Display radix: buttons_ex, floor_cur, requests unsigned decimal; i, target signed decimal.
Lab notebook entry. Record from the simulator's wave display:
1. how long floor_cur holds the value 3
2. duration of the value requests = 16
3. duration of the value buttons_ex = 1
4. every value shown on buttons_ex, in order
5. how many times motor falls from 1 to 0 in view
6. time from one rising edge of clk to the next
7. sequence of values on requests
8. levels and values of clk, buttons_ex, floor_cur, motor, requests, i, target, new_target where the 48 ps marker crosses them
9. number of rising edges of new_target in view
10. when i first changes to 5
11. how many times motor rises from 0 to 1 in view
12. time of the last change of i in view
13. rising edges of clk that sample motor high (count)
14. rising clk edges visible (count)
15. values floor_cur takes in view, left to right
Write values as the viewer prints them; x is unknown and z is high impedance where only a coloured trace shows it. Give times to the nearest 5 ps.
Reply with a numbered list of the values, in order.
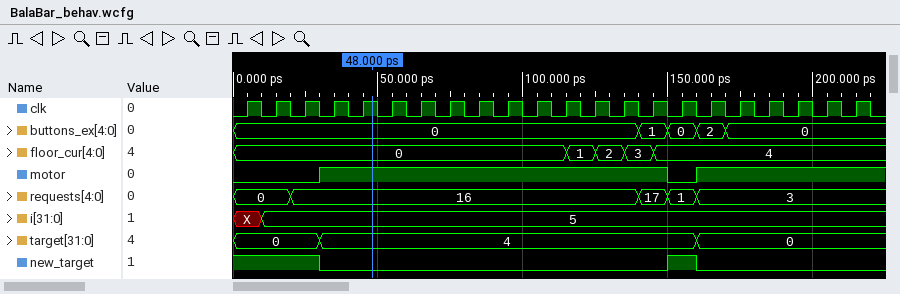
1. 10 ps
2. 120 ps
3. 10 ps
4. 0, 1, 0, 2, 0
5. 1
6. 10 ps
7. 0, 16, 17, 1, 3
8. clk=1, buttons_ex=0, floor_cur=0, motor=1, requests=16, i=5, target=4, new_target=0
9. 1
10. 10 ps
11. 2
12. 10 ps
13. 18
14. 22
15. 0, 1, 2, 3, 4
